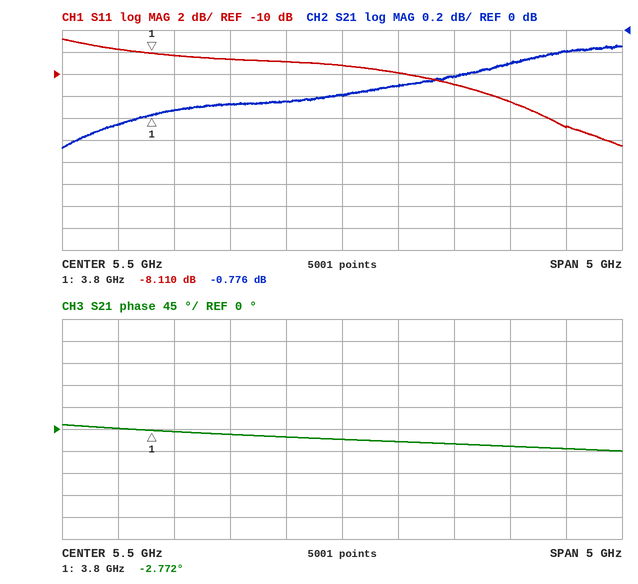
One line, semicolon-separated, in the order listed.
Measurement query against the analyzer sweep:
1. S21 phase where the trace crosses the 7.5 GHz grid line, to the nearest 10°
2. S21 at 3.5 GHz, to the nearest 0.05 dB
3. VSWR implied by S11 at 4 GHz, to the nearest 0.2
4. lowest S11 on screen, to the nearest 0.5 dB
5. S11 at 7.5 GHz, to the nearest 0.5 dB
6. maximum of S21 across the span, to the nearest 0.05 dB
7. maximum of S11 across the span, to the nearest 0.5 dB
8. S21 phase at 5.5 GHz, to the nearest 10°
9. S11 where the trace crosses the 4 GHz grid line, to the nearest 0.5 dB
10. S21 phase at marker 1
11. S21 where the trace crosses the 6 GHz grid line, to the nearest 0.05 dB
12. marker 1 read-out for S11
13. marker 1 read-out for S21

-40°; -0.85 dB; 2.2; -16.5 dB; -15.0 dB; -0.15 dB; -7.0 dB; -20°; -8.5 dB; -2.772°; -0.50 dB; -8.110 dB; -0.776 dB
